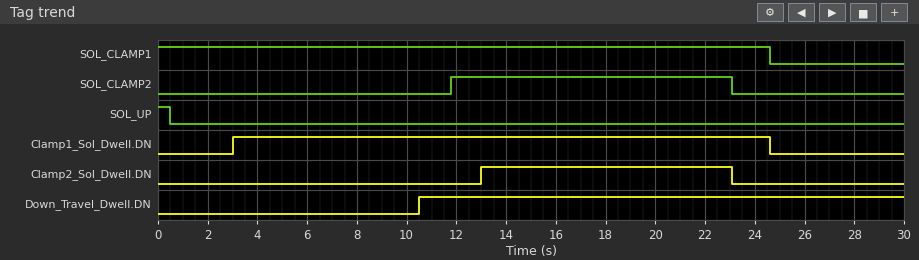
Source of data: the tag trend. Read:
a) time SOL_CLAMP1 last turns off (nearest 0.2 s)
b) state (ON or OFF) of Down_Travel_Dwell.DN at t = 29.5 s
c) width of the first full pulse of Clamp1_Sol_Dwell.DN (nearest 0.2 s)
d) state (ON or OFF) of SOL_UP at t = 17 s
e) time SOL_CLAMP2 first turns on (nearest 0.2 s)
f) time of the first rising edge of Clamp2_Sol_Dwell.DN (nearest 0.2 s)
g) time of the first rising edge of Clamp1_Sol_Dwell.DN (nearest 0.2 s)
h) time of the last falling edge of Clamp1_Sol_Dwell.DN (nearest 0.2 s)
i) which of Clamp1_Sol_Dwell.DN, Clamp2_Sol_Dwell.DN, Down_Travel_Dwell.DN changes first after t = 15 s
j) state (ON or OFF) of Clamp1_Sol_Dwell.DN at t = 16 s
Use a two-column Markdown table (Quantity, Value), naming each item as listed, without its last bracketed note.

| Quantity | Value |
|---|---|
| time SOL_CLAMP1 last turns off | 24.6 s |
| state (ON or OFF) of Down_Travel_Dwell.DN at t = 29.5 s | ON |
| width of the first full pulse of Clamp1_Sol_Dwell.DN | 21.6 s |
| state (ON or OFF) of SOL_UP at t = 17 s | OFF |
| time SOL_CLAMP2 first turns on | 11.8 s |
| time of the first rising edge of Clamp2_Sol_Dwell.DN | 13.0 s |
| time of the first rising edge of Clamp1_Sol_Dwell.DN | 3.0 s |
| time of the last falling edge of Clamp1_Sol_Dwell.DN | 24.6 s |
| which of Clamp1_Sol_Dwell.DN, Clamp2_Sol_Dwell.DN, Down_Travel_Dwell.DN changes first after t = 15 s | Clamp2_Sol_Dwell.DN |
| state (ON or OFF) of Clamp1_Sol_Dwell.DN at t = 16 s | ON |
